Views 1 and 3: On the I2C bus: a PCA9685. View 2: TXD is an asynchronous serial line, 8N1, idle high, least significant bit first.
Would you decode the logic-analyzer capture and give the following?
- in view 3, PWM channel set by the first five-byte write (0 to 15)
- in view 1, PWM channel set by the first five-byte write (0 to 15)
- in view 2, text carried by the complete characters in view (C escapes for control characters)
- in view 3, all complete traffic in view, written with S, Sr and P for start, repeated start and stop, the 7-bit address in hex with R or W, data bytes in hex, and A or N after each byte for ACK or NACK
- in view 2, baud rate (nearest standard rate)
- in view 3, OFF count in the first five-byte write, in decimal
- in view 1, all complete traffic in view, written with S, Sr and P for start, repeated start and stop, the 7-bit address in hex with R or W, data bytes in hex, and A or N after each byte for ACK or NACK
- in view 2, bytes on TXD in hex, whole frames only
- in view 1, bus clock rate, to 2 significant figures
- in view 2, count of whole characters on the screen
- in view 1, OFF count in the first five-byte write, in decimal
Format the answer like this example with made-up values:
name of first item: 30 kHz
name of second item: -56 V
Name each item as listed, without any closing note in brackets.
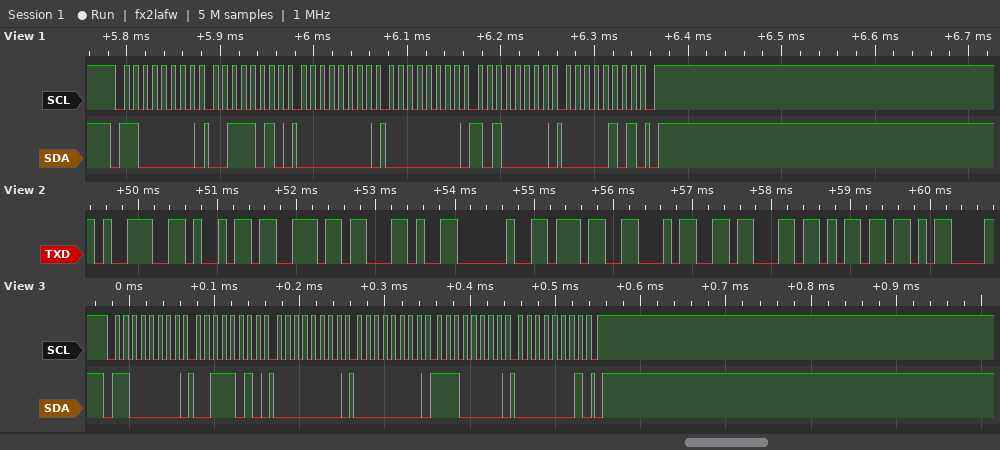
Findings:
in view 3, PWM channel set by the first five-byte write: 13
in view 1, PWM channel set by the first five-byte write: 13
in view 2, text carried by the complete characters in view: "9in, 74cm\r"
in view 3, all complete traffic in view, written with S, Sr and P for start, repeated start and stop, the 7-bit address in hex with R or W, data bytes in hex, and A or N after each byte for ACK or NACK: S 60W A 3A A 00 A 00 A E0 A 01 A P
in view 2, baud rate: 9600 baud
in view 3, OFF count in the first five-byte write, in decimal: 480
in view 1, all complete traffic in view, written with S, Sr and P for start, repeated start and stop, the 7-bit address in hex with R or W, data bytes in hex, and A or N after each byte for ACK or NACK: S 60W A 3A A 00 A 00 A A0 A 05 A P
in view 2, bytes on TXD in hex, whole frames only: 39 69 6E 2C 20 37 34 63 6D 0D
in view 1, bus clock rate, to 2 significant figures: 100 kHz
in view 2, count of whole characters on the screen: 10
in view 1, OFF count in the first five-byte write, in decimal: 1440
